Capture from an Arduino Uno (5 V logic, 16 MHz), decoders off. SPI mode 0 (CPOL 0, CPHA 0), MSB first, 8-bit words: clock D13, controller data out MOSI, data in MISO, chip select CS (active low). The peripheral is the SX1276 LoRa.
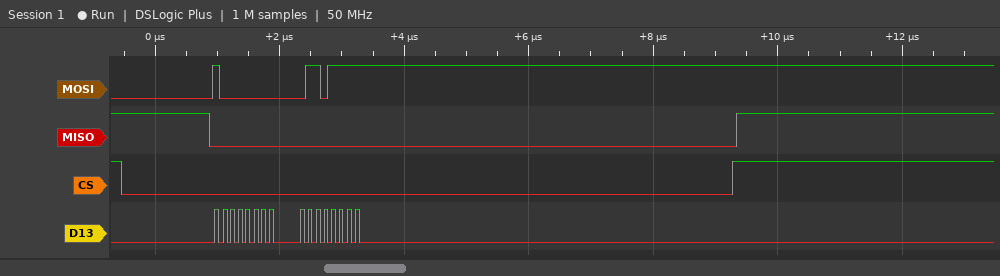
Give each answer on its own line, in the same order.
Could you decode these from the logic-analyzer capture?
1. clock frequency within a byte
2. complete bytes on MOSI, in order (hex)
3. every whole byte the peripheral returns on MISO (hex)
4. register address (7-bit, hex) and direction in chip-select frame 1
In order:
8 MHz
80 6F
00 00
0x00 write
